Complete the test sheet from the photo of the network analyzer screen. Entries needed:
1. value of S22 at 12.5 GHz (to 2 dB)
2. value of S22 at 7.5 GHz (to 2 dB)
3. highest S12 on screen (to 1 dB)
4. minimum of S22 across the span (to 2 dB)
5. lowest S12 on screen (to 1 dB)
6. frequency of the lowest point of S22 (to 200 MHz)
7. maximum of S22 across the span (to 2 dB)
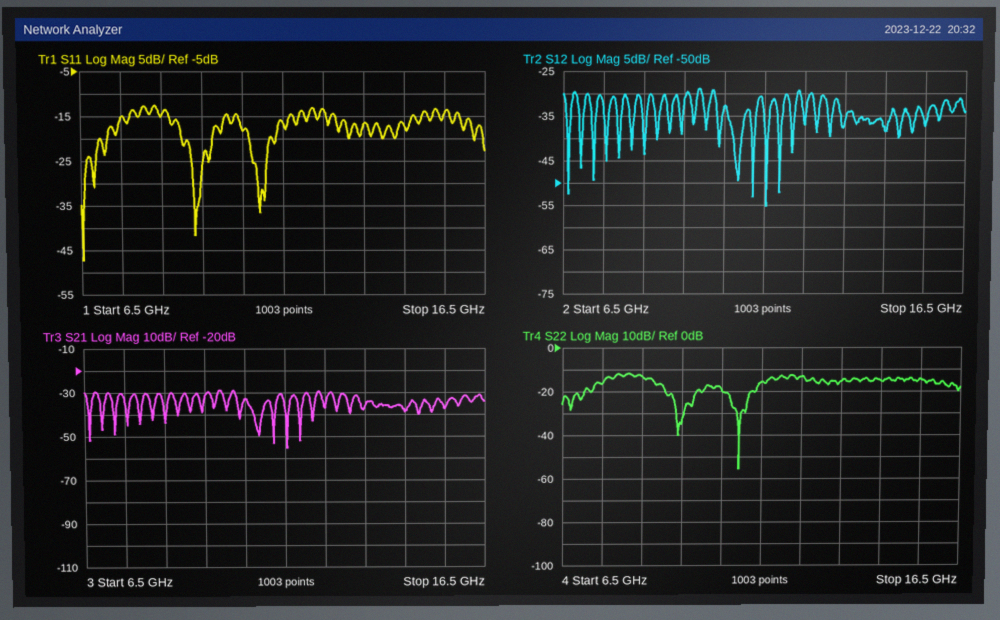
-14 dB
-16 dB
-29 dB
-56 dB
-55 dB
11.0 GHz
-12 dB
